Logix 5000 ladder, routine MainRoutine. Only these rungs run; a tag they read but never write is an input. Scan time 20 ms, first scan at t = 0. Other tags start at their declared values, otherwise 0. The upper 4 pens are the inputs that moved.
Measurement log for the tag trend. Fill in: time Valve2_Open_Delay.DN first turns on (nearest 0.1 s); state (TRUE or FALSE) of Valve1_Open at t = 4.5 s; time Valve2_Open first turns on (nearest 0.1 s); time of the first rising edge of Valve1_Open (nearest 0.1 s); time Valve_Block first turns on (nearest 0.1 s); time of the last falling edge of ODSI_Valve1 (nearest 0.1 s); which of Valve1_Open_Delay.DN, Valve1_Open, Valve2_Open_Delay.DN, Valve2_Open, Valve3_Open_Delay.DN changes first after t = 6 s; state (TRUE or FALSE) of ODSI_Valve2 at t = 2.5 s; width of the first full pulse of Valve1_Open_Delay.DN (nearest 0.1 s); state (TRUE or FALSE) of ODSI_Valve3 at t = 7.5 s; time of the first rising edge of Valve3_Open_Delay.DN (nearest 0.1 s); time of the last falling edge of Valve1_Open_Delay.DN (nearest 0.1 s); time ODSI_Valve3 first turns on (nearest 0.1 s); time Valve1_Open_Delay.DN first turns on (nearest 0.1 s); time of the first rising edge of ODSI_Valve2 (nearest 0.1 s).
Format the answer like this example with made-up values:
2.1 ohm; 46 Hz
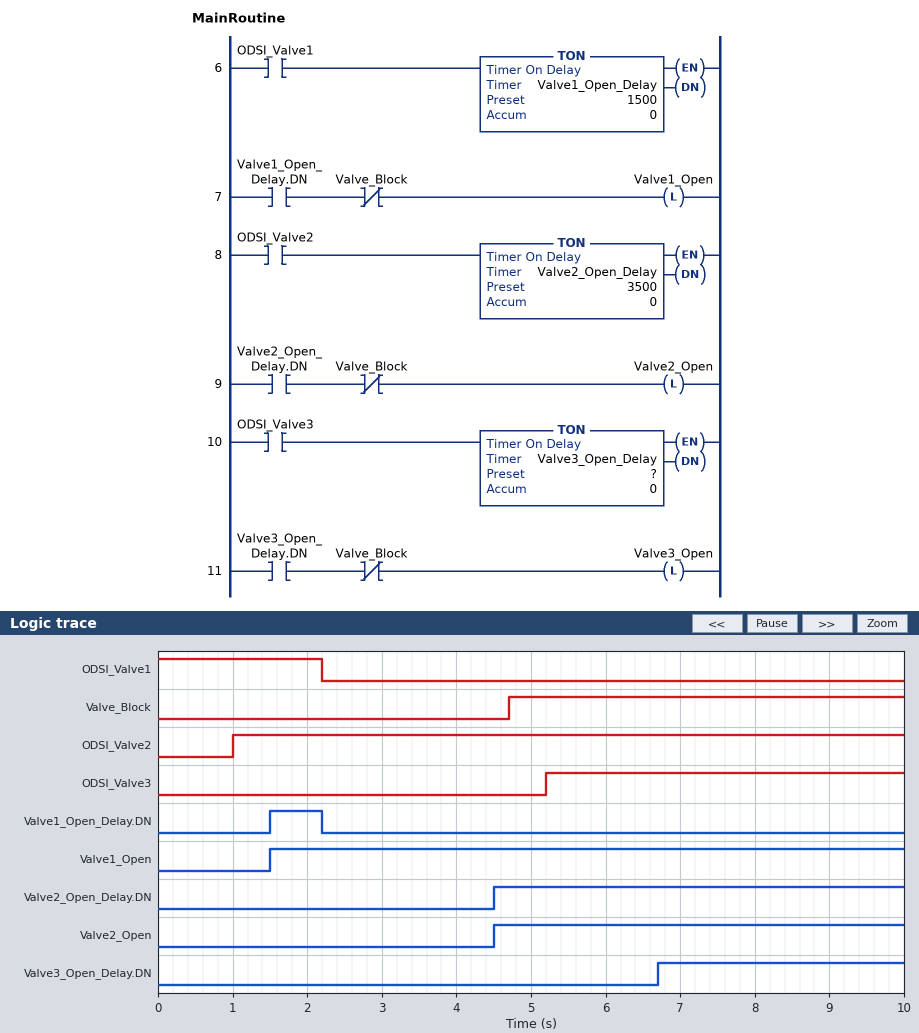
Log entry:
4.5 s; TRUE; 4.5 s; 1.5 s; 4.7 s; 2.2 s; Valve3_Open_Delay.DN; TRUE; 0.7 s; TRUE; 6.7 s; 2.2 s; 5.2 s; 1.5 s; 1.0 s
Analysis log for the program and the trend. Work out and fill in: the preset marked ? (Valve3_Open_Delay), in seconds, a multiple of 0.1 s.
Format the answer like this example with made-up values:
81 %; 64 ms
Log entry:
1.5 s
